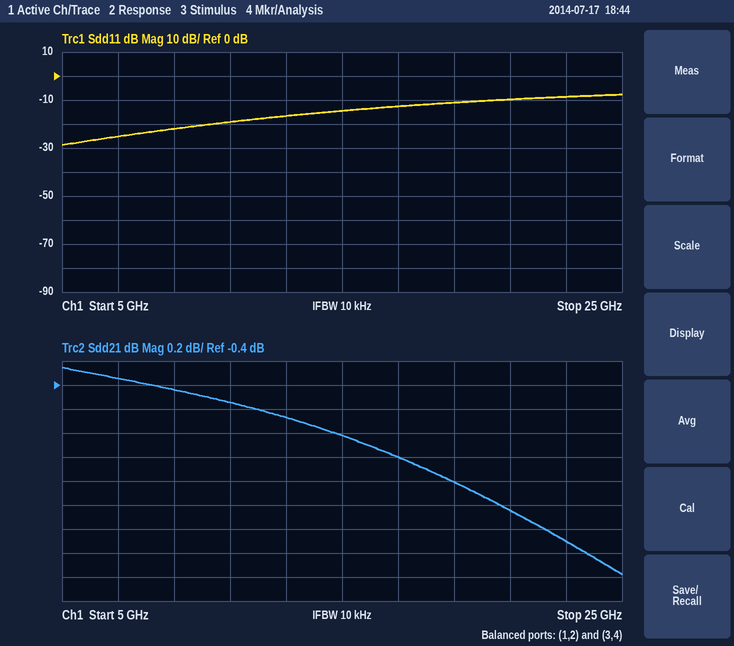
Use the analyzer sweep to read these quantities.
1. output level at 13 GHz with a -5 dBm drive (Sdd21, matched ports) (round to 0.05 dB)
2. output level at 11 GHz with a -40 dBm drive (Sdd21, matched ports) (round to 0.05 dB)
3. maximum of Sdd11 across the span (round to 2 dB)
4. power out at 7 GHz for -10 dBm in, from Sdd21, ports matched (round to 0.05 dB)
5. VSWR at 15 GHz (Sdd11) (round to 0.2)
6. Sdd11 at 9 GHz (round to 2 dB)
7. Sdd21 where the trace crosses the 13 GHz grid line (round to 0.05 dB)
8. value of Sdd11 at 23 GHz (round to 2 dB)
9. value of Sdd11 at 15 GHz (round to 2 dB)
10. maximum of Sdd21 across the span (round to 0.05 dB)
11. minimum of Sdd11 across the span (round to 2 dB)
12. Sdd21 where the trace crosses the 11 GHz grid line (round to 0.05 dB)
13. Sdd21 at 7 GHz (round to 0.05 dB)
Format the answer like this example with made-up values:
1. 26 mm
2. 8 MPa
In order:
1. -5.65 dBm
2. -40.55 dBm
3. -8 dB
4. -10.35 dBm
5. 1.4
6. -22 dB
7. -0.65 dB
8. -8 dB
9. -14 dB
10. -0.25 dB
11. -28 dB
12. -0.55 dB
13. -0.35 dB
